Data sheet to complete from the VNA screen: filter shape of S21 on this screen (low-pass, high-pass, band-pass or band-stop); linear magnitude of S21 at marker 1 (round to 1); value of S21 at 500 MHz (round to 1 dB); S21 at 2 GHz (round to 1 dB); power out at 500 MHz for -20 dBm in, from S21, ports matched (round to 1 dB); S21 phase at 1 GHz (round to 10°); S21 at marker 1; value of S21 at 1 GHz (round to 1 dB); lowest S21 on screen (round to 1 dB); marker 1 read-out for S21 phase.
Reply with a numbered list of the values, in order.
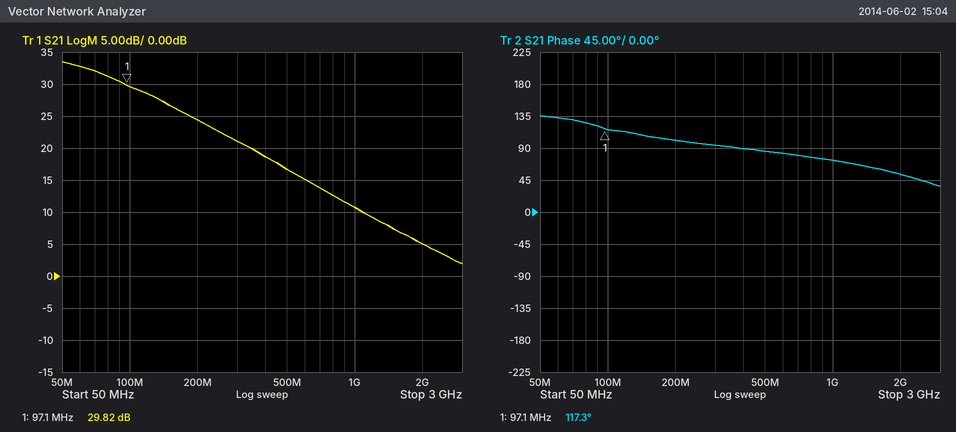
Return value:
1. low-pass
2. 31
3. 17 dB
4. 5 dB
5. -3 dBm
6. 70°
7. 29.82 dB
8. 11 dB
9. 2 dB
10. 117.3°
